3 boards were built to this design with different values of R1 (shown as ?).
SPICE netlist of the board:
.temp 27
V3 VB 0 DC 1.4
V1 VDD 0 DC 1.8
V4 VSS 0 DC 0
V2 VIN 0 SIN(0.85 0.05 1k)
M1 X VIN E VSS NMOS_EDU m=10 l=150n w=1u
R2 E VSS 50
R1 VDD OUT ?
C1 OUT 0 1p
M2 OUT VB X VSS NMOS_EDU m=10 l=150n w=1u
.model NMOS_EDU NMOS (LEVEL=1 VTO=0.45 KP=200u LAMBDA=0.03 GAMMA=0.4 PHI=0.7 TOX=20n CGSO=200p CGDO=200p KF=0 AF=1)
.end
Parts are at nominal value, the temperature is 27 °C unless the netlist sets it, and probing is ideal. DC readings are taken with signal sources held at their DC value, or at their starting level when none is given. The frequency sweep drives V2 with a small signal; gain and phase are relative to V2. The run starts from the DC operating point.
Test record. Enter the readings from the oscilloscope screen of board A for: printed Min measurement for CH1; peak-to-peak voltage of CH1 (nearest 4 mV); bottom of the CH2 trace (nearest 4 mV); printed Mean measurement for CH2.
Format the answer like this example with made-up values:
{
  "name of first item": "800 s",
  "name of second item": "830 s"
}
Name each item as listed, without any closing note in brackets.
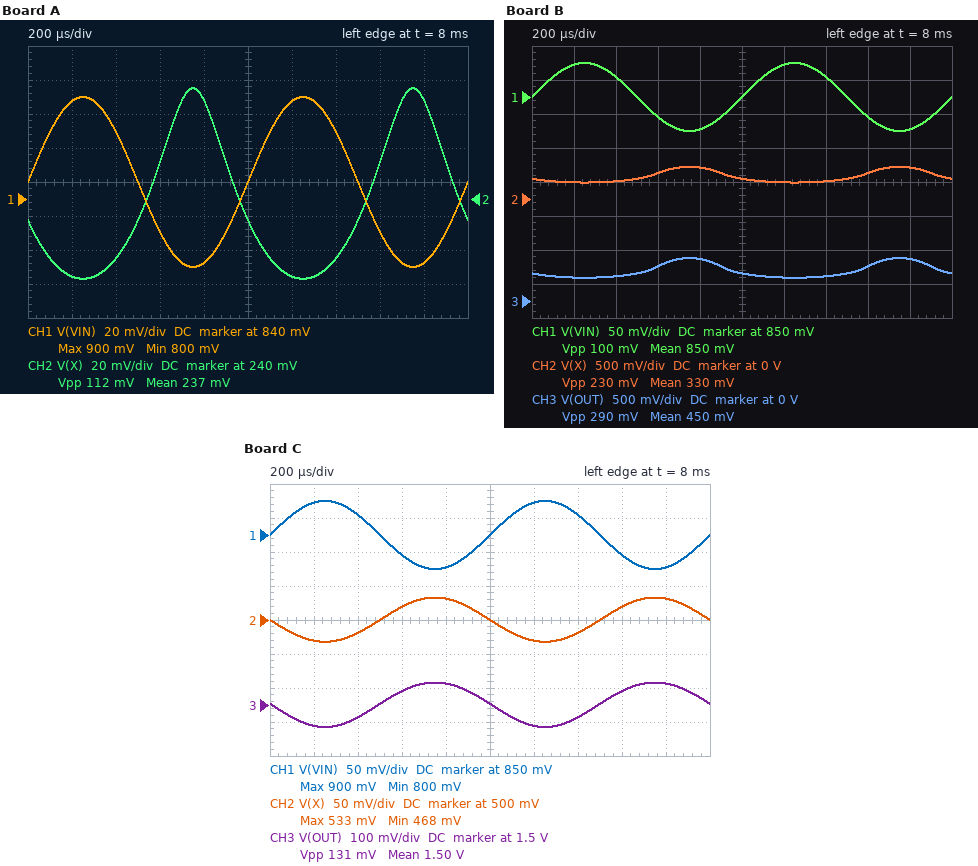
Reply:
{
  "printed Min measurement for CH1": "800 mV",
  "peak-to-peak voltage of CH1": "100 mV",
  "bottom of the CH2 trace": "192 mV",
  "printed Mean measurement for CH2": "237 mV"
}
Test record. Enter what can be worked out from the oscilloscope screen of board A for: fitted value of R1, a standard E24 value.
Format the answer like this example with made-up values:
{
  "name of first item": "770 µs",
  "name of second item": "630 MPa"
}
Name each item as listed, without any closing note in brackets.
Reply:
{
  "fitted value of R1, a standard E24 value": "2.2 kΩ"
}
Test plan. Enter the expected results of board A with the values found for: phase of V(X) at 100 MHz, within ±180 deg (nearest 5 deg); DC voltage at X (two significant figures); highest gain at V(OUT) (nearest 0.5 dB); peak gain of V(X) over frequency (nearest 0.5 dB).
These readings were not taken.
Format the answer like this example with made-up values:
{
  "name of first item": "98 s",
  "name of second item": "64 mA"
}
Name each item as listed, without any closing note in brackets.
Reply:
{
  "phase of V(X) at 100 MHz, within ±180 deg": "165 deg",
  "DC voltage at X": "230 mV",
  "highest gain at V(OUT)": "0 dB",
  "peak gain of V(X) over frequency": "-1.0 dB"
}
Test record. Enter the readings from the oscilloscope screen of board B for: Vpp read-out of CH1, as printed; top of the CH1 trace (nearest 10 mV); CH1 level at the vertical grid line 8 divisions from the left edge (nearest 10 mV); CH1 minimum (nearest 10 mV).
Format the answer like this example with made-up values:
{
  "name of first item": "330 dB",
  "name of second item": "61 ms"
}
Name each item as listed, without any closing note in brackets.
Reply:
{
  "Vpp read-out of CH1, as printed": "100 mV",
  "top of the CH1 trace": "900 mV",
  "CH1 level at the vertical grid line 8 divisions from the left edge": "820 mV",
  "CH1 minimum": "800 mV"
}
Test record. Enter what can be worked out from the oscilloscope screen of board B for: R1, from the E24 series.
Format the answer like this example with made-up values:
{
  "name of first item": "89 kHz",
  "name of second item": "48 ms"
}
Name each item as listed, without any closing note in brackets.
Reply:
{
  "R1, from the E24 series": "1.8 kΩ"
}
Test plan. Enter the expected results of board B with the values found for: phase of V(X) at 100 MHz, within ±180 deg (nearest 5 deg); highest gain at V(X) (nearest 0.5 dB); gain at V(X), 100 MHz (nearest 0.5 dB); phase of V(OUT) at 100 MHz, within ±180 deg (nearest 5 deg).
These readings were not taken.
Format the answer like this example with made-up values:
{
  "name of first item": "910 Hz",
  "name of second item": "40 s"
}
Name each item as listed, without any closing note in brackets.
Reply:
{
  "phase of V(X) at 100 MHz, within ±180 deg": "160 deg",
  "highest gain at V(X)": "4.5 dB",
  "gain at V(X), 100 MHz": "3.5 dB",
  "phase of V(OUT) at 100 MHz, within ±180 deg": "155 deg"
}
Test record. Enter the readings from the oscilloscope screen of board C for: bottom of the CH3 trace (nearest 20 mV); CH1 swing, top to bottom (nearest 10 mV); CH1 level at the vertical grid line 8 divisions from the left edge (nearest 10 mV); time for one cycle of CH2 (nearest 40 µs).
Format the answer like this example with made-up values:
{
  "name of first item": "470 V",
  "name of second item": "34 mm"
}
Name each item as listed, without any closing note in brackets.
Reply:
{
  "bottom of the CH3 trace": "1.44 V",
  "CH1 swing, top to bottom": "100 mV",
  "CH1 level at the vertical grid line 8 divisions from the left edge": "820 mV",
  "time for one cycle of CH2": "1.00 ms"
}
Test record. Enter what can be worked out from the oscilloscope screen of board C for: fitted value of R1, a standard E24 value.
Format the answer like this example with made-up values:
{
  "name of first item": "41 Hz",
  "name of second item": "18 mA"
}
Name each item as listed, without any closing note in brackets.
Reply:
{
  "fitted value of R1, a standard E24 value": "360 Ω"
}
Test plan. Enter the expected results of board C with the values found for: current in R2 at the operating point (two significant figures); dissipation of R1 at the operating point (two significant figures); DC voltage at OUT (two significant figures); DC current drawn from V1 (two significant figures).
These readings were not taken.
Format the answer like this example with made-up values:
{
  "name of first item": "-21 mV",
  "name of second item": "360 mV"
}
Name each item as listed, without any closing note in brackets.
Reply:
{
  "current in R2 at the operating point": "820 µA",
  "dissipation of R1 at the operating point": "240 µW",
  "DC voltage at OUT": "1.5 V",
  "DC current drawn from V1": "820 µA"
}
